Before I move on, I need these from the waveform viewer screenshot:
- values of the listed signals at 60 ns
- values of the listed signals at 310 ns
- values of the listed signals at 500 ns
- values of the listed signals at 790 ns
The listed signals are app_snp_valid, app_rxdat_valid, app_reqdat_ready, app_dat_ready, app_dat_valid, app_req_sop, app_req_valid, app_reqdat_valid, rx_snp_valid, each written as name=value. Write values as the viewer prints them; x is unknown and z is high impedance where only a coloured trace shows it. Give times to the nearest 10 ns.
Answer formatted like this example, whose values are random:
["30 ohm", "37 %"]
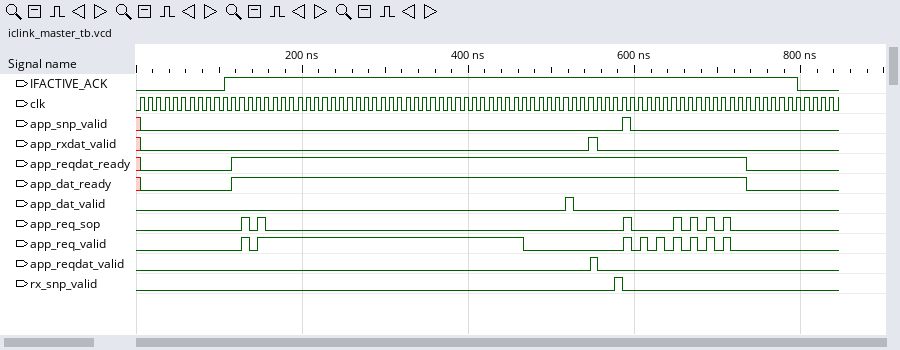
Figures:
["app_snp_valid=0, app_rxdat_valid=0, app_reqdat_ready=0, app_dat_ready=0, app_dat_valid=0, app_req_sop=0, app_req_valid=0, app_reqdat_valid=0, rx_snp_valid=0", "app_snp_valid=0, app_rxdat_valid=0, app_reqdat_ready=1, app_dat_ready=1, app_dat_valid=0, app_req_sop=0, app_req_valid=1, app_reqdat_valid=0, rx_snp_valid=0", "app_snp_valid=0, app_rxdat_valid=0, app_reqdat_ready=1, app_dat_ready=1, app_dat_valid=0, app_req_sop=0, app_req_valid=0, app_reqdat_valid=0, rx_snp_valid=0", "app_snp_valid=0, app_rxdat_valid=0, app_reqdat_ready=0, app_dat_ready=0, app_dat_valid=0, app_req_sop=0, app_req_valid=0, app_reqdat_valid=0, rx_snp_valid=0"]
